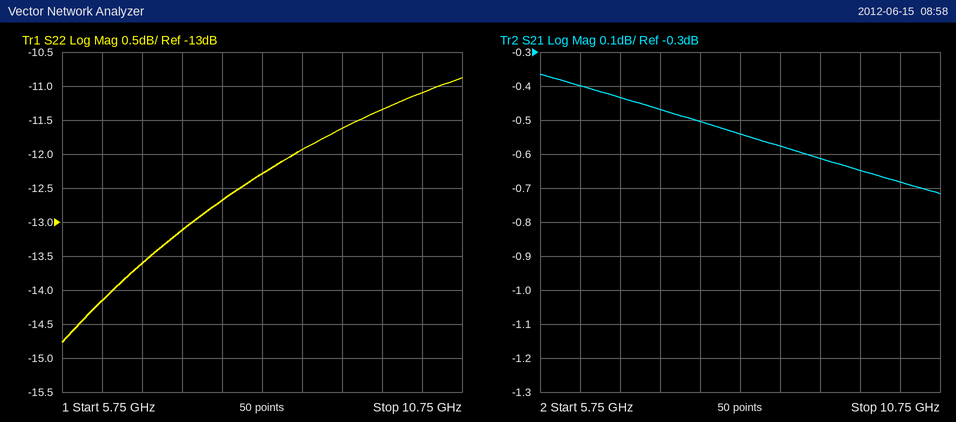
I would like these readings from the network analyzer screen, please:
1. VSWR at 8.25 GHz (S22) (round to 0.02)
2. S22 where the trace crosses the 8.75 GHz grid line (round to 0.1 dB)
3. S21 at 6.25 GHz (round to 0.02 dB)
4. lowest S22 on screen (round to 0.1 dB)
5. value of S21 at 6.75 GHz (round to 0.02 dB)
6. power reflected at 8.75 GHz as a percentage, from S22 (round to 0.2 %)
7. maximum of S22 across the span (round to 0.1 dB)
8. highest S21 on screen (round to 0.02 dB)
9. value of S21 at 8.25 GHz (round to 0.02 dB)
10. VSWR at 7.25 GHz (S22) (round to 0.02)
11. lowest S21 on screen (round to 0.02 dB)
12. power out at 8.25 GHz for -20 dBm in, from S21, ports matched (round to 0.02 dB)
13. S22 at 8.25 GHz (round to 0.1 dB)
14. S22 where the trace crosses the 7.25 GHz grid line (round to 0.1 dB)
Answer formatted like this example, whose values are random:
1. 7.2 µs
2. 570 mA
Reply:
1. 1.64
2. -11.9 dB
3. -0.40 dB
4. -14.8 dB
5. -0.44 dB
6. 6.4 %
7. -10.9 dB
8. -0.36 dB
9. -0.54 dB
10. 1.56
11. -0.72 dB
12. -20.54 dBm
13. -12.3 dB
14. -13.1 dB
